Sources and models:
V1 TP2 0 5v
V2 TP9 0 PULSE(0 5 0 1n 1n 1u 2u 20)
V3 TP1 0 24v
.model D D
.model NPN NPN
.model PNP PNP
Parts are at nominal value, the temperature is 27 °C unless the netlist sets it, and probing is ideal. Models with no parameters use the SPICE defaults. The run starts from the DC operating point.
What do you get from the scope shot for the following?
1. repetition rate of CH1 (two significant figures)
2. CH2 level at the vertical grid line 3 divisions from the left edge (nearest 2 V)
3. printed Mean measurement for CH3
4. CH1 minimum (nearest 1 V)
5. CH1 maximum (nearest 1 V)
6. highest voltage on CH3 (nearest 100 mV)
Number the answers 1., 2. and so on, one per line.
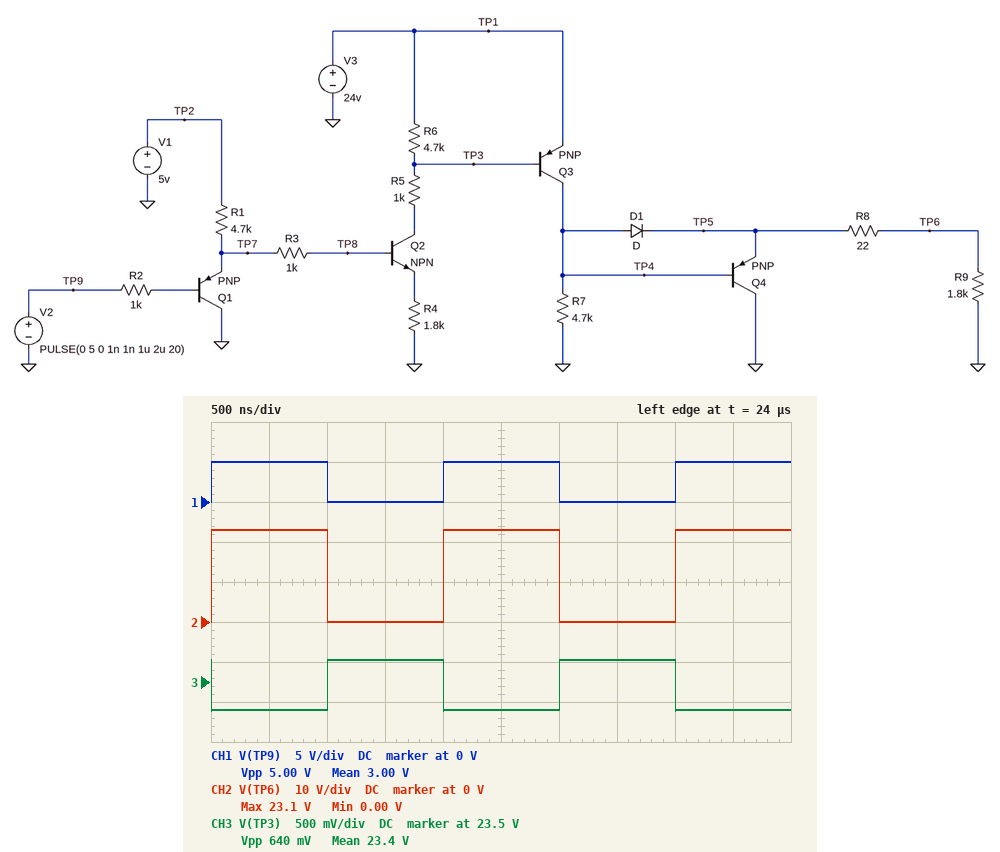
1. 500 kHz
2. 0 V
3. 23.4 V
4. 0 V
5. 5 V
6. 23.8 V
